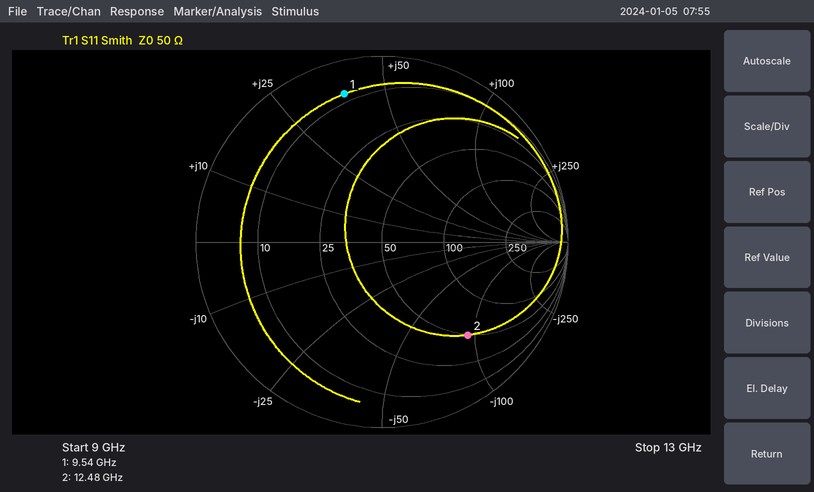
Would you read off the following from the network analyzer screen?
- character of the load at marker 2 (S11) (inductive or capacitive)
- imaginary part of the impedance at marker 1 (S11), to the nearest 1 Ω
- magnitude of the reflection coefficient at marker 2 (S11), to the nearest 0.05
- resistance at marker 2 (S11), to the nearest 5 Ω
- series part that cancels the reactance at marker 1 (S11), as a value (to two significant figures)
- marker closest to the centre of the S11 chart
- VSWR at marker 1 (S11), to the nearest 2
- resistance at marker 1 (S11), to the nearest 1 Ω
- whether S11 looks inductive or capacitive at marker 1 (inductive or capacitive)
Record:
capacitive
+38 Ω
0.70
50 Ω
440 fF
marker 2
10
8 Ω
inductive
